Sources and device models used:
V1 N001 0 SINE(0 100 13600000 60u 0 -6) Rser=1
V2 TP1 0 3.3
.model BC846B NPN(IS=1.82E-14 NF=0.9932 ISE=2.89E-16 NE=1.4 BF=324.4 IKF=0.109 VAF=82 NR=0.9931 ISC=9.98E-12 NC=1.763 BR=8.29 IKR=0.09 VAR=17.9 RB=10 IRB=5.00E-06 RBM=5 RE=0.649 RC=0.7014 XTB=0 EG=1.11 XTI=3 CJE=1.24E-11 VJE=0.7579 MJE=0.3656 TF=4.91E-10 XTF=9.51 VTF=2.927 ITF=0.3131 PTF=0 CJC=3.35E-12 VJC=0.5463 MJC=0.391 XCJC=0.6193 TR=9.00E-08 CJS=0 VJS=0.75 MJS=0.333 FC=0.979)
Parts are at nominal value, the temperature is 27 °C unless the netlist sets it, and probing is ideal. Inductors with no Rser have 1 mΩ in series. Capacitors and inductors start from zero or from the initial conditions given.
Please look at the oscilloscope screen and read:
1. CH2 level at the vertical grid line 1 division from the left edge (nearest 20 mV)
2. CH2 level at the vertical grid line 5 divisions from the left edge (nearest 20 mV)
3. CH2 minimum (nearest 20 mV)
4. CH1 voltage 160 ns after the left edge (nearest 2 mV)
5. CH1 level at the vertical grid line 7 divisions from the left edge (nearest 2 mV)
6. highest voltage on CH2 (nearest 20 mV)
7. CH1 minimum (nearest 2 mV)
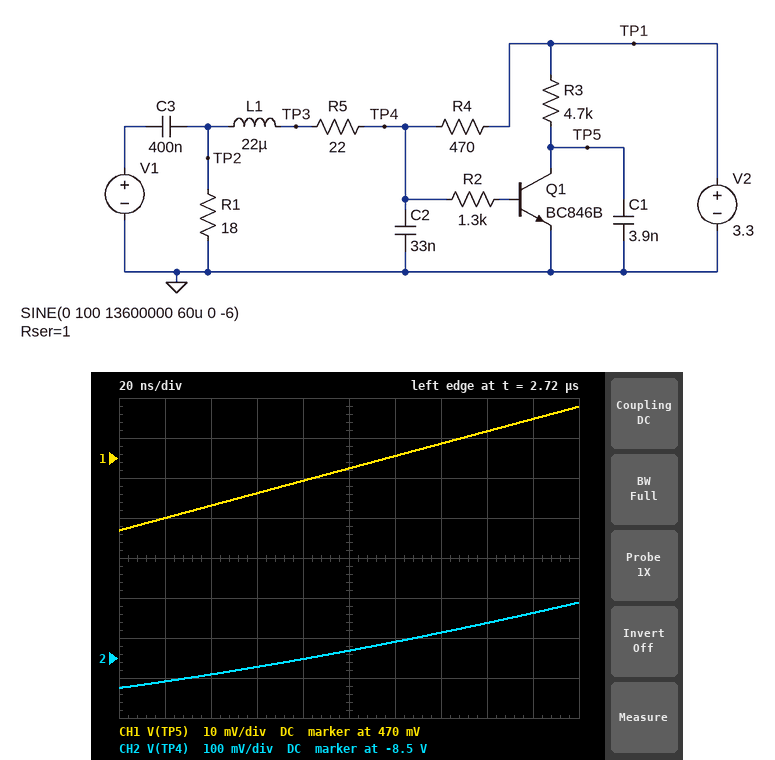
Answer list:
-8.56 V
-8.48 V
-8.58 V
476 mV
474 mV
-8.36 V
452 mV
